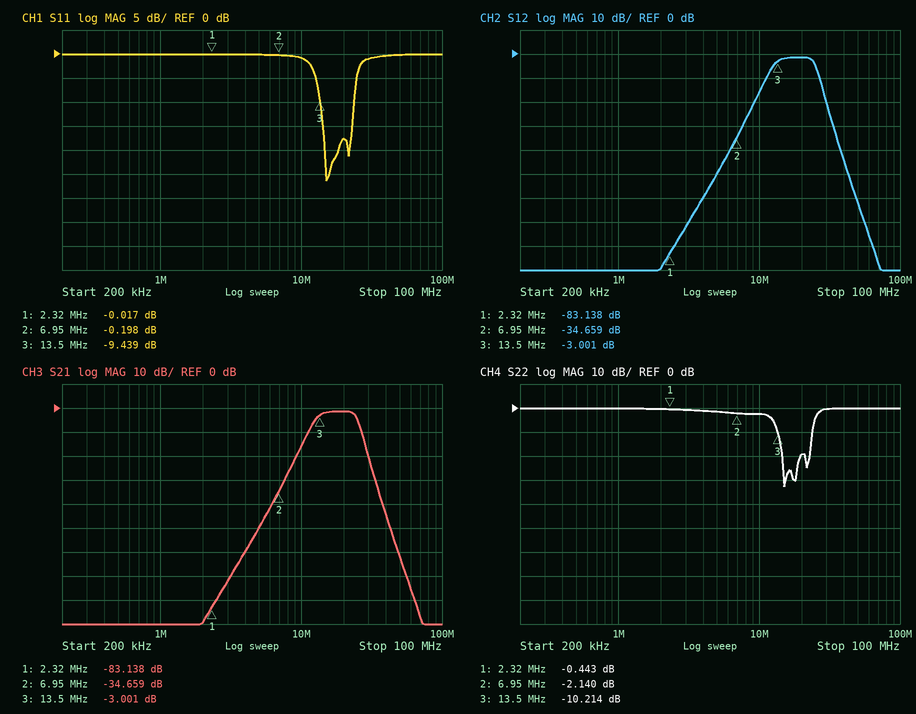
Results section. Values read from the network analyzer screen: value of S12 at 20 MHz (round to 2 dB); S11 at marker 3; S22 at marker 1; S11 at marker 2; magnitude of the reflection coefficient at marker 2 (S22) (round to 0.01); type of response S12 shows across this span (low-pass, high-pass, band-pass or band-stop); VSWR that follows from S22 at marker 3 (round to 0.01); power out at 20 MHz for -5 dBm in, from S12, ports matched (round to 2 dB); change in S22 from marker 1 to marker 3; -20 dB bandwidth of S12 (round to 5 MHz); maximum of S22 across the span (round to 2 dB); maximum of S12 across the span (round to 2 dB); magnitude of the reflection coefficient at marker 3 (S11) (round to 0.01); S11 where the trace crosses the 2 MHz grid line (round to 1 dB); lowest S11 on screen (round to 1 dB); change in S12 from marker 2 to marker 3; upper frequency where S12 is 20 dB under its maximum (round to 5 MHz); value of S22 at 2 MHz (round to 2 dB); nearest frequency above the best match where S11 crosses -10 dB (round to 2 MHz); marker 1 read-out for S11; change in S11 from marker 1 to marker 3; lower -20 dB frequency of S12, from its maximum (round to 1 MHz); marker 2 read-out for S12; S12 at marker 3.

-2 dB
-9.439 dB
-0.443 dB
-0.198 dB
0.78
band-pass
1.89
-6 dBm
-9.771 dB
20 MHz
0 dB
-2 dB
0.34
0 dB
-26 dB
31.658 dB
30 MHz
0 dB
24 MHz
-0.017 dB
-9.422 dB
9 MHz
-34.659 dB
-3.001 dB
